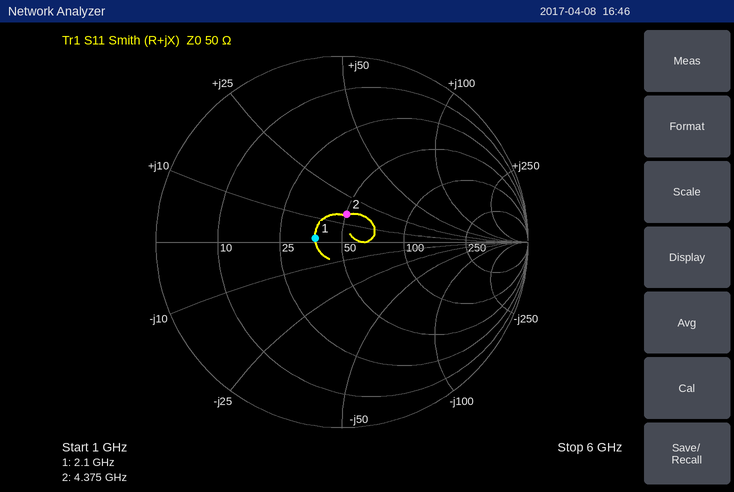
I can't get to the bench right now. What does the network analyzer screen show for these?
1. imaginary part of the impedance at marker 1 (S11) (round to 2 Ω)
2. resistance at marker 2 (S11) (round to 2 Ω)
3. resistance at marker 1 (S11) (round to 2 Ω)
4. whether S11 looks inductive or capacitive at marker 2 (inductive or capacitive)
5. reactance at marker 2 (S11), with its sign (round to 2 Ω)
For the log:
+2 Ω
50 Ω
38 Ω
inductive
+16 Ω
